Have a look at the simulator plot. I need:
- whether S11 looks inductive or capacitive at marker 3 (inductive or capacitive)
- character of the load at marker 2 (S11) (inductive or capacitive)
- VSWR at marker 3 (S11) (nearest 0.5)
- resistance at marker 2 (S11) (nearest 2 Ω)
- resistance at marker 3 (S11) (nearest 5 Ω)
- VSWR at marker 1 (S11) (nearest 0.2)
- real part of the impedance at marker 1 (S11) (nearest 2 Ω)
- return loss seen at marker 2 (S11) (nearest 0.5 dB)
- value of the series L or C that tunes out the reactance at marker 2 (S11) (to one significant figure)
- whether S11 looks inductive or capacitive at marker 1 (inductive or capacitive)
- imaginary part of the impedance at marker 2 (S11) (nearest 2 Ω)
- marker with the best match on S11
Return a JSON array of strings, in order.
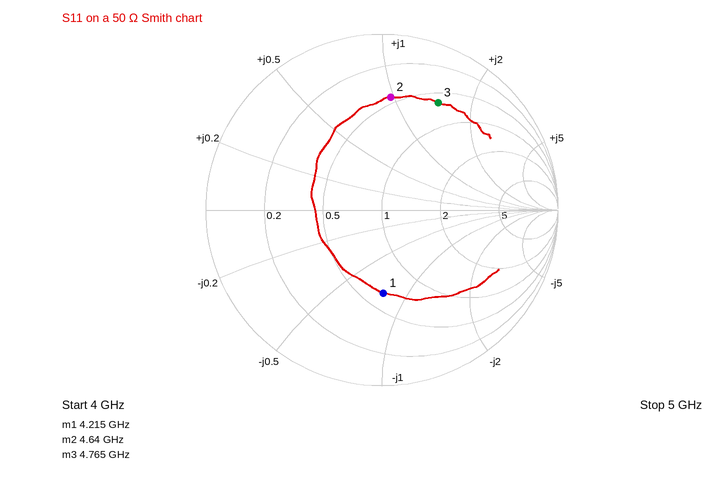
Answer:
["inductive", "inductive", "5.5", "22 Ω", "30 Ω", "2.8", "32 Ω", "4.0 dB", "700 fF", "capacitive", "+48 Ω", "marker 1"]
